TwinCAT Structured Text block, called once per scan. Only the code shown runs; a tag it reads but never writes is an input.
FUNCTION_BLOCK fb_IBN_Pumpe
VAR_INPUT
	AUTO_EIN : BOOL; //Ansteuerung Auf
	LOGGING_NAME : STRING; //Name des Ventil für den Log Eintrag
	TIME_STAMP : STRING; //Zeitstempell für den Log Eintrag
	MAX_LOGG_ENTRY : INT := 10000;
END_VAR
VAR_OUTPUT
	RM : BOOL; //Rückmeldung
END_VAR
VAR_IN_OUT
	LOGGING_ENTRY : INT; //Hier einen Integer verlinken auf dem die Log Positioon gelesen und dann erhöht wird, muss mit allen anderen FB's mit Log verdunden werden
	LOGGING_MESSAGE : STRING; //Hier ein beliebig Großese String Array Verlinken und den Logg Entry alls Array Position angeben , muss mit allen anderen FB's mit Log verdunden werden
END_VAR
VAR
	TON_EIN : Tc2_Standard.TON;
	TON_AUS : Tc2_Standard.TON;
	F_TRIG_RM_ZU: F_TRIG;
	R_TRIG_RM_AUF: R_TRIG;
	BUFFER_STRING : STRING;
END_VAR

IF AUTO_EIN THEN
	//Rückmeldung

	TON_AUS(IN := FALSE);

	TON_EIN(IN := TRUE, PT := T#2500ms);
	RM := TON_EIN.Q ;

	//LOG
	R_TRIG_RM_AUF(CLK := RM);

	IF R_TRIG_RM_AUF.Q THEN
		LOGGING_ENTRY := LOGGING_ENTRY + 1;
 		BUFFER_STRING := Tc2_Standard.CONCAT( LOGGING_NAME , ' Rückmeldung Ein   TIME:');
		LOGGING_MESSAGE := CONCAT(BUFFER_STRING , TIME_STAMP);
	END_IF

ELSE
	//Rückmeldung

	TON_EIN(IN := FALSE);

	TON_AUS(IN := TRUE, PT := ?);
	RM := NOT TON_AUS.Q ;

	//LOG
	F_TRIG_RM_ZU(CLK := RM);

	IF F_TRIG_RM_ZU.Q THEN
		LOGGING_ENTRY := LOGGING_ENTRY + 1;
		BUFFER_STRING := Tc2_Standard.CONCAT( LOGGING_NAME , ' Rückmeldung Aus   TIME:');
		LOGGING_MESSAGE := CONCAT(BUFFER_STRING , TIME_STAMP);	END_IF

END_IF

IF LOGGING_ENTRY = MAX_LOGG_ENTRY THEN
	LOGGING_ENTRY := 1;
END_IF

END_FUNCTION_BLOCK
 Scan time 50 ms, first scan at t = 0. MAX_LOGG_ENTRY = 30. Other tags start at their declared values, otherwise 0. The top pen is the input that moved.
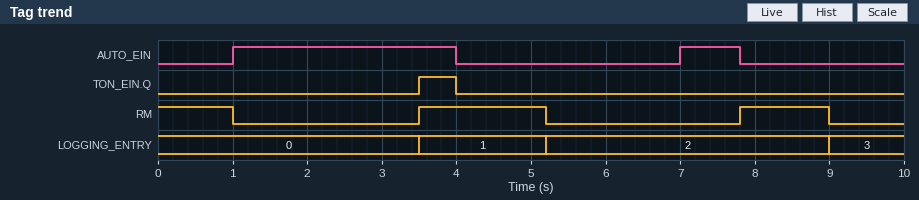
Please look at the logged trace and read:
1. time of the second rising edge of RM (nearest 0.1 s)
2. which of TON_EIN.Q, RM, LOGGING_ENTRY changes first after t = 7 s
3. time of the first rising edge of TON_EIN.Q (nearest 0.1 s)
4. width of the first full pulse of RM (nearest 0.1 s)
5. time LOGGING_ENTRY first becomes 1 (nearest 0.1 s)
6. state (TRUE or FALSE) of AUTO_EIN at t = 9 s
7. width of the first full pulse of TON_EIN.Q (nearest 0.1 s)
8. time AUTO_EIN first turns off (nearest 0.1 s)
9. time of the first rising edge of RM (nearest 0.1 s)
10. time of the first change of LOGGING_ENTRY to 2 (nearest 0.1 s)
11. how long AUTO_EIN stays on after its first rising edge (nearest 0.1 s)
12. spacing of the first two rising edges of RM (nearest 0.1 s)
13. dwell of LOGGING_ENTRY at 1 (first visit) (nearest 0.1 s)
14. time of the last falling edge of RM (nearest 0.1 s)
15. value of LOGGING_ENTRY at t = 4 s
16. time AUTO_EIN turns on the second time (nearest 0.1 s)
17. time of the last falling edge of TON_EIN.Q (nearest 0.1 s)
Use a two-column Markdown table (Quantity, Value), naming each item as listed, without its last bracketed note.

| Quantity | Value |
|---|---|
| time of the second rising edge of RM | 7.8 s |
| which of TON_EIN.Q, RM, LOGGING_ENTRY changes first after t = 7 s | RM |
| time of the first rising edge of TON_EIN.Q | 3.5 s |
| width of the first full pulse of RM | 1.7 s |
| time LOGGING_ENTRY first becomes 1 | 3.5 s |
| state (TRUE or FALSE) of AUTO_EIN at t = 9 s | FALSE |
| width of the first full pulse of TON_EIN.Q | 0.5 s |
| time AUTO_EIN first turns off | 4.0 s |
| time of the first rising edge of RM | 3.5 s |
| time of the first change of LOGGING_ENTRY to 2 | 5.2 s |
| how long AUTO_EIN stays on after its first rising edge | 3.0 s |
| spacing of the first two rising edges of RM | 4.3 s |
| dwell of LOGGING_ENTRY at 1 (first visit) | 1.7 s |
| time of the last falling edge of RM | 9.0 s |
| value of LOGGING_ENTRY at t = 4 s | 1 |
| time AUTO_EIN turns on the second time | 7.0 s |
| time of the last falling edge of TON_EIN.Q | 4.0 s |
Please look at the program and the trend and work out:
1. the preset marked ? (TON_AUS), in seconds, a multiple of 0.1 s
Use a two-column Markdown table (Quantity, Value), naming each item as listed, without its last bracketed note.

| Quantity | Value |
|---|---|
| the preset marked ? (TON_AUS), in seconds, a multiple of 0.1 s | 1.2 s |
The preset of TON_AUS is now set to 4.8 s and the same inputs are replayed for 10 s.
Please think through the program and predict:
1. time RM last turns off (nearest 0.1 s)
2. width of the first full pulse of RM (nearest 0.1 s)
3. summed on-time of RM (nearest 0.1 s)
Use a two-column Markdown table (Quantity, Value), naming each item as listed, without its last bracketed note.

| Quantity | Value |
|---|---|
| time RM last turns off | 7.0 s |
| width of the first full pulse of RM | 3.5 s |
| summed on-time of RM | 6.7 s |
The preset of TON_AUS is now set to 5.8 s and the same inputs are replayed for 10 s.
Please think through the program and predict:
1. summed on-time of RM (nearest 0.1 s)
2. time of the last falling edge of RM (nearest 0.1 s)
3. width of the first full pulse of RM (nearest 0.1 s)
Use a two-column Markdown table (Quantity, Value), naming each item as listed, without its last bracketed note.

| Quantity | Value |
|---|---|
| summed on-time of RM | 6.7 s |
| time of the last falling edge of RM | 7.0 s |
| width of the first full pulse of RM | 3.5 s |
